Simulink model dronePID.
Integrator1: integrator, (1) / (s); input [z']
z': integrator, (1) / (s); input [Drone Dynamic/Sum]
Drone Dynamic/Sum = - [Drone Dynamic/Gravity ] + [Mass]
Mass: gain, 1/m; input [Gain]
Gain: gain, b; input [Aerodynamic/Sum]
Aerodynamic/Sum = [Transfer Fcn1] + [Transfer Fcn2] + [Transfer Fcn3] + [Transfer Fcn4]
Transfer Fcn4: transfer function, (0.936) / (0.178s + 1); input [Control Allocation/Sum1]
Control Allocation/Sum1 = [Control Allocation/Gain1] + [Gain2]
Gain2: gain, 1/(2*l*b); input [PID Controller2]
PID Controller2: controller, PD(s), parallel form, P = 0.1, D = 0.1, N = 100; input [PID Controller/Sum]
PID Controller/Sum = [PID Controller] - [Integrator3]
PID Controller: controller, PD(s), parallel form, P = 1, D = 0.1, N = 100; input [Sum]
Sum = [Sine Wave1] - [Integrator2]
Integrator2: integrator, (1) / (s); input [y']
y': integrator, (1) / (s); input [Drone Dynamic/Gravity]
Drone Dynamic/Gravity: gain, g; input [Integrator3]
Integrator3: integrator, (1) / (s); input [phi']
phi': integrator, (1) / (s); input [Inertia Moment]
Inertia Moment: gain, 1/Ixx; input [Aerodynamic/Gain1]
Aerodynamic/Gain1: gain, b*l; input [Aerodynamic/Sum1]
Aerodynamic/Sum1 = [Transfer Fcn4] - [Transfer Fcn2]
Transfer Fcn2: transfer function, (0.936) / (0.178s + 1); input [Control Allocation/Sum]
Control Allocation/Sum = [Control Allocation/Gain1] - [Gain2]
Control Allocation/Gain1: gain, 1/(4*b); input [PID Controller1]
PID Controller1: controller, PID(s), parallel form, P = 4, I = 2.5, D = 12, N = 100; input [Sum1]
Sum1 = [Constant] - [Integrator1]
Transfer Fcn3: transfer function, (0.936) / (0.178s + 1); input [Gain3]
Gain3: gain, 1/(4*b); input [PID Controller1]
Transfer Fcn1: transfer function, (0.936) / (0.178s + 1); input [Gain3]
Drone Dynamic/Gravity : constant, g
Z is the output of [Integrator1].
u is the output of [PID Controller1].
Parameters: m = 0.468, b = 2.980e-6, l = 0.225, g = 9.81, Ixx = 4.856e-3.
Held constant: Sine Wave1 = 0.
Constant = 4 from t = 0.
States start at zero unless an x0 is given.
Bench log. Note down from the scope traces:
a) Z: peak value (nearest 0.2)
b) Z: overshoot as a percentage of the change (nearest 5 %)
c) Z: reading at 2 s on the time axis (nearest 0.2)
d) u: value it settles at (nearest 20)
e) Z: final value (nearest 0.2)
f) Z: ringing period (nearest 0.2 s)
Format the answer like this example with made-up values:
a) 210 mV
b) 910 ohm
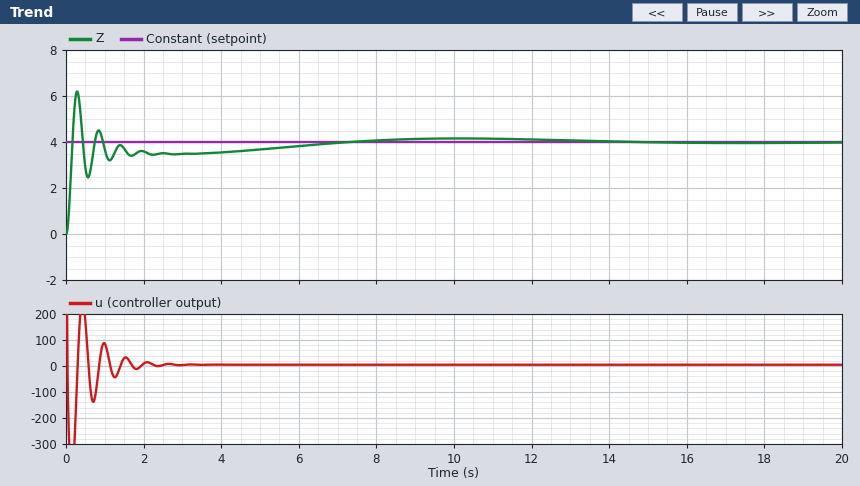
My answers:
a) 6.2
b) 55 %
c) 3.6
d) 0
e) 4.0
f) 0.6 s
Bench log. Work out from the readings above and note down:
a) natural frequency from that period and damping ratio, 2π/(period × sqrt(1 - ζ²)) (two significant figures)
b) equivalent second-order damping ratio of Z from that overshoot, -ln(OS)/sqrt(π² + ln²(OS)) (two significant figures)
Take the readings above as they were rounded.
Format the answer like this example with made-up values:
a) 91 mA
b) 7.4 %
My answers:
a) 11 rad/s
b) 0.19
